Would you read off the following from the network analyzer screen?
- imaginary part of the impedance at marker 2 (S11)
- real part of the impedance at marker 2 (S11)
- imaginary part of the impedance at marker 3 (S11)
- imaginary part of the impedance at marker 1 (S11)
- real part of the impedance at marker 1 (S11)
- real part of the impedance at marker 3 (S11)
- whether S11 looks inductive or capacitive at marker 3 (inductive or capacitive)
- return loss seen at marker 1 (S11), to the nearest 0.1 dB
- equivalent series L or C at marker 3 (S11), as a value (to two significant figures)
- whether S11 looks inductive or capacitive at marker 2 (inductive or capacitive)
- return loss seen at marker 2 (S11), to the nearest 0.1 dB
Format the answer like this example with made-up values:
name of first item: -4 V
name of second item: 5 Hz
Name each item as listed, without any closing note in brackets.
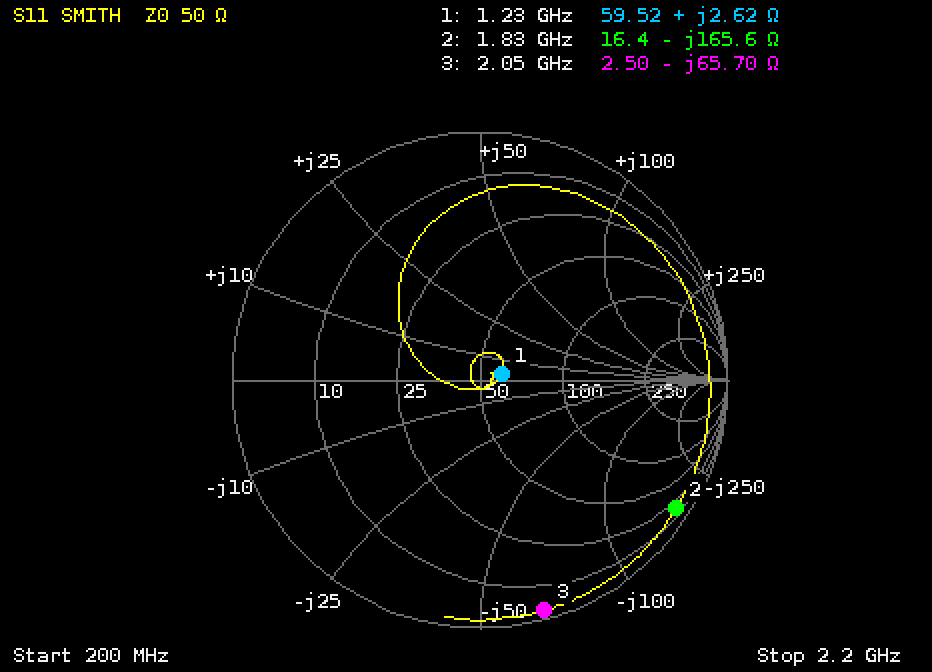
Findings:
imaginary part of the impedance at marker 2: -165.6 Ω
real part of the impedance at marker 2: 16.4 Ω
imaginary part of the impedance at marker 3: -65.70 Ω
imaginary part of the impedance at marker 1: +2.62 Ω
real part of the impedance at marker 1: 59.52 Ω
real part of the impedance at marker 3: 2.50 Ω
whether S11 looks inductive or capacitive at marker 3: capacitive
return loss seen at marker 1 (S11), to the nearest 0.1 dB: 20.9 dB
equivalent series L or C at marker 3 (S11), as a value: 1.2 pF
whether S11 looks inductive or capacitive at marker 2: capacitive
return loss seen at marker 2 (S11), to the nearest 0.1 dB: 0.5 dB
